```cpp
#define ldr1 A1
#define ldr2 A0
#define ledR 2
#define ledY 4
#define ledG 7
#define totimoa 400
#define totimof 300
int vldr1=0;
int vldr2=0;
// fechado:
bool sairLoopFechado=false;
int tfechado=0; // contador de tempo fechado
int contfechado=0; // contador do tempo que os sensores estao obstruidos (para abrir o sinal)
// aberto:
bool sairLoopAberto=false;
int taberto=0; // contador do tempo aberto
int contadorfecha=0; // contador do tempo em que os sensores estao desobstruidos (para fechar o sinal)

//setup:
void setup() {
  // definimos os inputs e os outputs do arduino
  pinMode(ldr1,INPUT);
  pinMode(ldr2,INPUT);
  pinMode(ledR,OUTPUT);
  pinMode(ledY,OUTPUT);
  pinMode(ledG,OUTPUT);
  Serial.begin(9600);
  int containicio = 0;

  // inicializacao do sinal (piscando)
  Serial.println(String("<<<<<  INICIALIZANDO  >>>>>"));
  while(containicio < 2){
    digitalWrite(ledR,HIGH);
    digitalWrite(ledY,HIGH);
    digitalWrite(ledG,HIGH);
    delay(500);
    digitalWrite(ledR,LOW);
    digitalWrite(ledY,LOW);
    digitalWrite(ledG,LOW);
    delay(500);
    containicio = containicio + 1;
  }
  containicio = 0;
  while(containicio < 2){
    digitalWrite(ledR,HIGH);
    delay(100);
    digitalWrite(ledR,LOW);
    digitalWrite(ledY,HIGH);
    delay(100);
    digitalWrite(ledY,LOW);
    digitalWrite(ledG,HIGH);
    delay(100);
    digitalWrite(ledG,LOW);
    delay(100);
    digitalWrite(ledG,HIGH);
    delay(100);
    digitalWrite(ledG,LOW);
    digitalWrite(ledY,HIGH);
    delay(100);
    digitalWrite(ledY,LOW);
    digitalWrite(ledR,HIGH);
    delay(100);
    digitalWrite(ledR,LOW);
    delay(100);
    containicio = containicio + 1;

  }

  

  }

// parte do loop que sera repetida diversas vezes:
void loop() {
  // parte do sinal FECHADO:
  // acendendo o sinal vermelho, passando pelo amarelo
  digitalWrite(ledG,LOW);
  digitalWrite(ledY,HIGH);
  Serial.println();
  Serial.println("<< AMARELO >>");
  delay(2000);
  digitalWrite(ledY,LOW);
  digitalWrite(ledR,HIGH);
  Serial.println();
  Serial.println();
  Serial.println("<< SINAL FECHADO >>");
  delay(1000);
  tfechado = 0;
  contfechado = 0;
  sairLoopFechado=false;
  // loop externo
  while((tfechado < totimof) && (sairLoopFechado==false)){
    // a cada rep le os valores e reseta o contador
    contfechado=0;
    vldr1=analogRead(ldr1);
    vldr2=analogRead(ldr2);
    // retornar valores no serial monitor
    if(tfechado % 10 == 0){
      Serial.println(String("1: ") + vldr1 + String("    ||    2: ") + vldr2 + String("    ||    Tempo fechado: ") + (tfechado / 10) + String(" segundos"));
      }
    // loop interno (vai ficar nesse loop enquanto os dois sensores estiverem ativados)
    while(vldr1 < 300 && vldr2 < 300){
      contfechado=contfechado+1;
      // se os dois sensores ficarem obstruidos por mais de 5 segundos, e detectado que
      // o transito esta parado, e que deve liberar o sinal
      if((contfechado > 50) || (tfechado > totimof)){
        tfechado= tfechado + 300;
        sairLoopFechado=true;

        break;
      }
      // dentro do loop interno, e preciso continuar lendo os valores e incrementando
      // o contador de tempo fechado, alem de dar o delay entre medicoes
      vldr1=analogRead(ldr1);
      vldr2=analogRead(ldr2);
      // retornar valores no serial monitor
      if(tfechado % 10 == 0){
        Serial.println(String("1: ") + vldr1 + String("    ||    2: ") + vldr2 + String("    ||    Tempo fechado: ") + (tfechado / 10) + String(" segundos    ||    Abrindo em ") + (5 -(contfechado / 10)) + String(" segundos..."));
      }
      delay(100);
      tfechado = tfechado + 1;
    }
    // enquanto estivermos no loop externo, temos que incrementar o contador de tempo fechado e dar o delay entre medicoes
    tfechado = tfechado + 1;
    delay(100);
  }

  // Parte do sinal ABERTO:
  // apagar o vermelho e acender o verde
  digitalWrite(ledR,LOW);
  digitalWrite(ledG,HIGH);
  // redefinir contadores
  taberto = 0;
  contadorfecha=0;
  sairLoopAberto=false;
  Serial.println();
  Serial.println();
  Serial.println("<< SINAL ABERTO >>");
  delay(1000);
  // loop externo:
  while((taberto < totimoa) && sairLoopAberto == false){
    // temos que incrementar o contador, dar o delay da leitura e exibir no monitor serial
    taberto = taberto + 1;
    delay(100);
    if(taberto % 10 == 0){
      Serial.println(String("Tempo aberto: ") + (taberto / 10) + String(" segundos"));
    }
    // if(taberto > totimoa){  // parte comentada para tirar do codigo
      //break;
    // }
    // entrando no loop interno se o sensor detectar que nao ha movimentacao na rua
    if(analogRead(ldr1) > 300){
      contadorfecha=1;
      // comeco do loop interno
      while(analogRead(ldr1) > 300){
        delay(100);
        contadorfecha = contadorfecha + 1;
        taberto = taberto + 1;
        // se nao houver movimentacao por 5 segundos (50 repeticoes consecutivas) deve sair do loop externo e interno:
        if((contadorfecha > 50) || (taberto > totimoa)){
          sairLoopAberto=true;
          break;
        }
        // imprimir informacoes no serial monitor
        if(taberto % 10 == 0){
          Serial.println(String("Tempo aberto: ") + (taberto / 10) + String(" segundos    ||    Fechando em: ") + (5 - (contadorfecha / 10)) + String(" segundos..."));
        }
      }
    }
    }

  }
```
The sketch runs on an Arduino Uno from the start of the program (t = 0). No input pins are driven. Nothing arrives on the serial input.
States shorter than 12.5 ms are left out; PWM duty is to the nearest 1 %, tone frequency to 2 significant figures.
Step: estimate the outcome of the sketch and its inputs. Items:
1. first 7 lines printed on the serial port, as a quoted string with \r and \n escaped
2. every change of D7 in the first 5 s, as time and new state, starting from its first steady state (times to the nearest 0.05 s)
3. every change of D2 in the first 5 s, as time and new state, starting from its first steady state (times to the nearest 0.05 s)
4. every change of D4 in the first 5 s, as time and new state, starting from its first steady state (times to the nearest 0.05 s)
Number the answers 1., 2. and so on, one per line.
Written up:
1. "<<<<<  INICIALIZANDO  >>>>>\r\n\r\n<< AMARELO >>\r\n\r\n\r\n<< SINAL FECHADO >>\r\n1: 0    ||    2: 0    ||    Tempo fechado: 0 segundos\r\n"
2. 0 s high; 0.5 s low; 1 s high; 1.5 s low; 2.2 s high; 2.3 s low; 2.4 s high; 2.5 s low; 3 s high; 3.1 s low; 3.2 s high; 3.3 s low
3. 0 s high; 0.5 s low; 1 s high; 1.5 s low; 2 s high; 2.1 s low; 2.6 s high; 2.7 s low; 2.8 s high; 2.9 s low; 3.4 s high; 3.5 s low
4. 0 s high; 0.5 s low; 1 s high; 1.5 s low; 2.1 s high; 2.2 s low; 2.5 s high; 2.6 s low; 2.9 s high; 3 s low; 3.3 s high; 3.4 s low; 3.6 s high
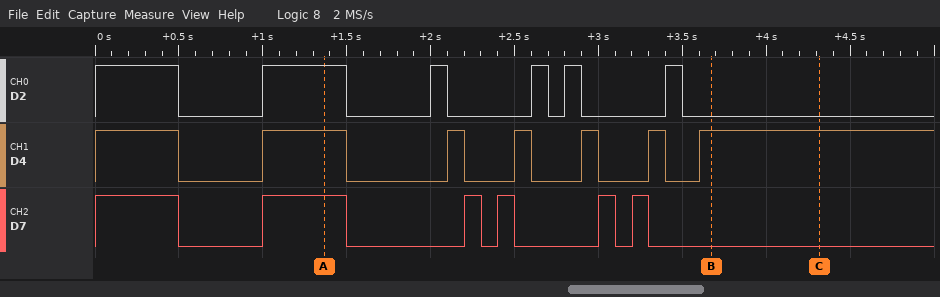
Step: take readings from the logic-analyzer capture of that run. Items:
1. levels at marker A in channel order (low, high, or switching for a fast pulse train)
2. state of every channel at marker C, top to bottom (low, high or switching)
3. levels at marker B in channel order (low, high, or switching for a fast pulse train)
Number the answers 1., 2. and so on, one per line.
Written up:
1. D2 high, D4 high, D7 high
2. D2 low, D4 high, D7 low
3. D2 low, D4 high, D7 low
